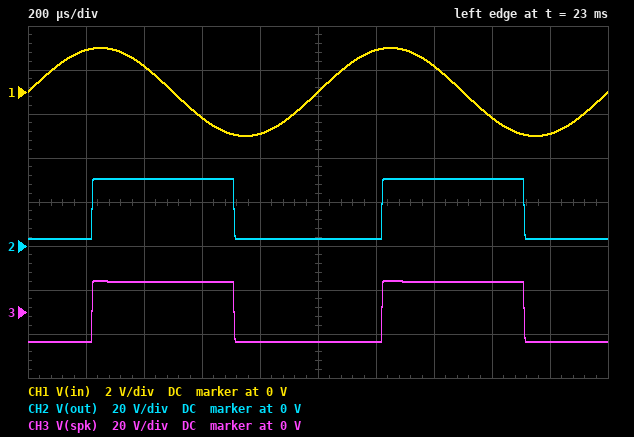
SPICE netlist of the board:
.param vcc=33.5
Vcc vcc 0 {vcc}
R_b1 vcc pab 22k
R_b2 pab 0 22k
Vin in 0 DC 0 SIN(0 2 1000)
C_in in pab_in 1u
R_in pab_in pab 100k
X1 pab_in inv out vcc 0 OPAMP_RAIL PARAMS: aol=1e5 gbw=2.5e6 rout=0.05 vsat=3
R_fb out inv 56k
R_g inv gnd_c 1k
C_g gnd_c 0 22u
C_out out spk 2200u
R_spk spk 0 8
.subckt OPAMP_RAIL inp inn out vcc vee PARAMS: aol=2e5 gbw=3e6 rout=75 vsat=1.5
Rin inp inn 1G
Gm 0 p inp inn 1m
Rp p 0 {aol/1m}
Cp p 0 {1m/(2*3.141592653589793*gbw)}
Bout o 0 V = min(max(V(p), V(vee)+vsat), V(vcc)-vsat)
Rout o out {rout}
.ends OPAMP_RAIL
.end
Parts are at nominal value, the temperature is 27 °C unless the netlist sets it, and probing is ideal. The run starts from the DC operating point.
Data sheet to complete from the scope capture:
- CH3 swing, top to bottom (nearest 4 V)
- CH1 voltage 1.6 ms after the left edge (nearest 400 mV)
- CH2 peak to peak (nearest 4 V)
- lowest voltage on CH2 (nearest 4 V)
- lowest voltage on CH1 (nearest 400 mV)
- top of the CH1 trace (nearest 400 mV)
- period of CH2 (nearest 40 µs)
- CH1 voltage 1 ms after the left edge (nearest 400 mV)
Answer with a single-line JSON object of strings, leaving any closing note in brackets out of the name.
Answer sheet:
{"CH3 swing, top to bottom": "28 V", "CH1 voltage 1.6 ms after the left edge": "-1.2 V", "CH2 peak to peak": "28 V", "lowest voltage on CH2": "4 V", "lowest voltage on CH1": "-2.0 V", "top of the CH1 trace": "2.0 V", "period of CH2": "1.00 ms", "CH1 voltage 1 ms after the left edge": "0 V"}
